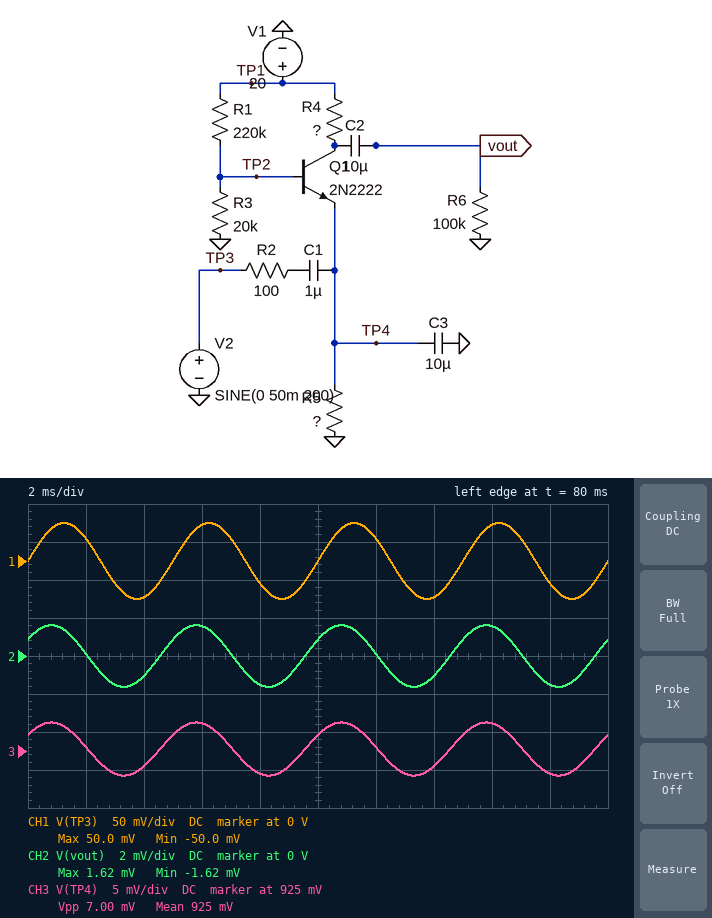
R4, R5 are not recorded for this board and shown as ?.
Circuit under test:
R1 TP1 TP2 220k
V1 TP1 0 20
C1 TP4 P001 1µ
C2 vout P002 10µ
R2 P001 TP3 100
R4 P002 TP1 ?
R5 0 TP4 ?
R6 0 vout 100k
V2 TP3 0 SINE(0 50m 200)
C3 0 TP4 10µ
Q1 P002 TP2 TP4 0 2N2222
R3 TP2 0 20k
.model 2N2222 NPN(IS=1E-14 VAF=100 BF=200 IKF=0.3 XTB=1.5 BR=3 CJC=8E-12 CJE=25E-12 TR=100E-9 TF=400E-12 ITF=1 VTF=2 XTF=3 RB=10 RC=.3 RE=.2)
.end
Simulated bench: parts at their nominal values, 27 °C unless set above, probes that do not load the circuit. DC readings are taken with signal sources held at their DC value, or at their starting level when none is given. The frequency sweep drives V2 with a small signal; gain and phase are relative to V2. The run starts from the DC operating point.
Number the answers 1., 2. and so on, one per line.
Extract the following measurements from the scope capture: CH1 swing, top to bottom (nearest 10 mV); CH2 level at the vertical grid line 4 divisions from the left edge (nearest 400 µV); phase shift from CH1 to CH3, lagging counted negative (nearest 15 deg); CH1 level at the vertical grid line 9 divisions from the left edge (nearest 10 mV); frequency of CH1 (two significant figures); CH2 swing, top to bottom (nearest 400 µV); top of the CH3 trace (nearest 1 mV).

1. 100 mV
2. -1.6 mV
3. 30 deg
4. -30 mV
5. 200 Hz
6. 3.2 mV
7. 929 mV
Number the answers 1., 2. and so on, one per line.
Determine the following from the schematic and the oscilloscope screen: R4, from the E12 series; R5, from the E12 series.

1. 47 Ω
2. 820 Ω
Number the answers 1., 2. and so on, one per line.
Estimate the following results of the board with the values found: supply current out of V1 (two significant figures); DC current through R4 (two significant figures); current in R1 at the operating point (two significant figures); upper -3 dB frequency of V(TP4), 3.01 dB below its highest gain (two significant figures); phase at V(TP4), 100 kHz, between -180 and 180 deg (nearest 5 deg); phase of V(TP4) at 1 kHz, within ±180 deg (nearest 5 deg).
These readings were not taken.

1. 1.2 mA
2. 1.1 mA
3. 84 µA
4. 2.1 kHz
5. -90 deg
6. -20 deg
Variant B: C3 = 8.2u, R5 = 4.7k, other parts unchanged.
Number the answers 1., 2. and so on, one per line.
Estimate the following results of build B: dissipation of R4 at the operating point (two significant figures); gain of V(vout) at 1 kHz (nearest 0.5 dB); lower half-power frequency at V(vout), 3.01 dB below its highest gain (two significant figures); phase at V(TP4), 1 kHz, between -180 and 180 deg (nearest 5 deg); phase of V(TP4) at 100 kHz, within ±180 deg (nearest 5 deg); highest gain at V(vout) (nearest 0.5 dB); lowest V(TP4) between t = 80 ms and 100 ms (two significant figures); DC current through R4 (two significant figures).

1. 2.3 µW
2. -33.0 dB
3. 84 Hz
4. -25 deg
5. -90 deg
6. -32.0 dB
7. 1.0 V
8. 220 µA
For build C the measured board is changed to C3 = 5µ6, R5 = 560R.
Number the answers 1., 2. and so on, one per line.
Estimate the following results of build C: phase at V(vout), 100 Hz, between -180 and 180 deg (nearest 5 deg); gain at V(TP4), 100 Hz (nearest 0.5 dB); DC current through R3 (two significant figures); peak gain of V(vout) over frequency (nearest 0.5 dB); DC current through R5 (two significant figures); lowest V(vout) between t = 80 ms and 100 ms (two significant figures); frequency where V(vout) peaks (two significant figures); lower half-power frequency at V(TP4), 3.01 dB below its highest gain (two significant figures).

1. 70 deg
2. -26.5 dB
3. 77 µA
4. -24.0 dB
5. 1.6 mA
6. -2.1 mV
7. 750 Hz
8. 230 Hz
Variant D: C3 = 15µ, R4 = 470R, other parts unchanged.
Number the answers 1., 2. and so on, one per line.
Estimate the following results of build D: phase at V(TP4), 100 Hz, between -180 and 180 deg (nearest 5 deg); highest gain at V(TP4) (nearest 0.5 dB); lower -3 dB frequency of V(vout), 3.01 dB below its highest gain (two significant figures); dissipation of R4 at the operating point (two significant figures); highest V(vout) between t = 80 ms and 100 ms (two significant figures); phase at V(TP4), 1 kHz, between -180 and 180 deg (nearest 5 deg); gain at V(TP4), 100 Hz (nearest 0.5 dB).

1. 45 deg
2. -24.5 dB
3. 98 Hz
4. 590 µW
5. 12 mV
6. -25 deg
7. -27.5 dB
